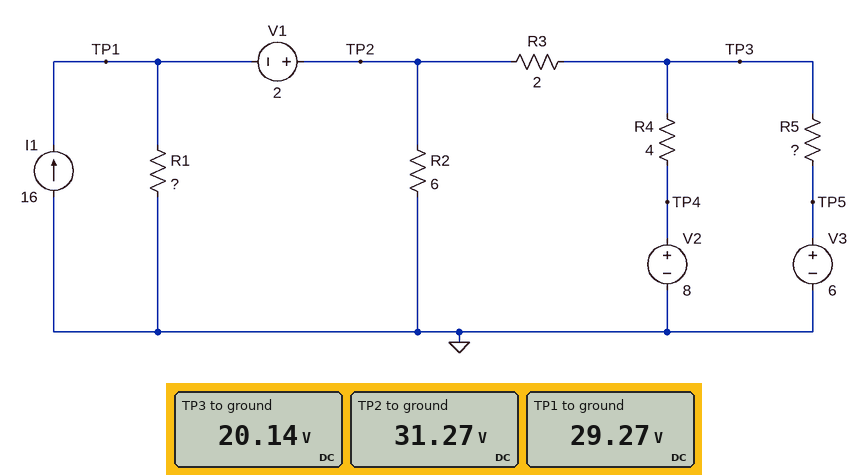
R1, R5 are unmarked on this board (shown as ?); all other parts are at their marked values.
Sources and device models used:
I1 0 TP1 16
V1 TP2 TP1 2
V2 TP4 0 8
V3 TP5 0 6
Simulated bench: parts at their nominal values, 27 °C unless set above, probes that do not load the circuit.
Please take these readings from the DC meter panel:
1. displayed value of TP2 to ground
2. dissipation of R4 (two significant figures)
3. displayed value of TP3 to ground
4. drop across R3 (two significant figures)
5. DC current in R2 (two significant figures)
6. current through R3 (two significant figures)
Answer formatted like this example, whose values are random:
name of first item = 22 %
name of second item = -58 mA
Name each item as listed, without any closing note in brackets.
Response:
displayed value of TP2 to ground = 31.27 V
dissipation of R4 = 37 W
displayed value of TP3 to ground = 20.14 V
drop across R3 = 11 V
DC current in R2 = 5.2 A
current through R3 = 5.6 A
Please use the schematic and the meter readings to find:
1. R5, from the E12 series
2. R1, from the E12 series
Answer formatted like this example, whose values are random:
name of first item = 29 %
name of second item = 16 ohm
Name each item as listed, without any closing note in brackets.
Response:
R5, from the E12 series = 5.6 Ω
R1, from the E12 series = 5.6 Ω
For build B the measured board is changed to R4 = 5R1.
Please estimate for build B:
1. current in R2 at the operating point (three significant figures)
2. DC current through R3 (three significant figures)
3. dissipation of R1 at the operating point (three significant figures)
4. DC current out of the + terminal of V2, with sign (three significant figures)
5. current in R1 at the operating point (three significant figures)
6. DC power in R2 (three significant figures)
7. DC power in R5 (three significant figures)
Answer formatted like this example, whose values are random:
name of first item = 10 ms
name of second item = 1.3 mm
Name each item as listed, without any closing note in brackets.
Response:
current in R2 at the operating point = 5.32 A
DC current through R3 = 5.33 A
dissipation of R1 at the operating point = 160 W
DC current out of the + terminal of V2, with sign = -2.60 A
current in R1 at the operating point = 5.35 A
DC power in R2 = 170 W
DC power in R5 = 41.7 W
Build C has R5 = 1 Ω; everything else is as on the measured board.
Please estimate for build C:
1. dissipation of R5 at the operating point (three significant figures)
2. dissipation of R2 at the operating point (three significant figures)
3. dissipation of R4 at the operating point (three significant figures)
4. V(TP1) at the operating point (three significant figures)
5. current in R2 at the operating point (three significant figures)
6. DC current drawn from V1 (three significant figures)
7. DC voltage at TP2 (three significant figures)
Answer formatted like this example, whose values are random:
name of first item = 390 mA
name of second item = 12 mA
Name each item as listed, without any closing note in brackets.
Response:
dissipation of R5 at the operating point = 37.9 W
dissipation of R2 at the operating point = 117 W
dissipation of R4 at the operating point = 4.32 W
V(TP1) at the operating point = 24.5 V
current in R2 at the operating point = 4.42 A
DC current drawn from V1 = 11.6 A
DC voltage at TP2 = 26.5 V
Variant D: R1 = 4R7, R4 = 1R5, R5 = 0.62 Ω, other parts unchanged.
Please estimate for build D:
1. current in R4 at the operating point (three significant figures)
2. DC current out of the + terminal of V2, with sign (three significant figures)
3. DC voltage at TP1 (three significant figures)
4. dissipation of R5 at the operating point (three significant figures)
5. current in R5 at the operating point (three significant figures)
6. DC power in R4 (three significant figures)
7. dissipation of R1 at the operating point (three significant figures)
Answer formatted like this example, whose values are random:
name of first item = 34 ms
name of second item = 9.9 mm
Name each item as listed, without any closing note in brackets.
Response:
current in R4 at the operating point = 1.17 A
DC current out of the + terminal of V2, with sign = -1.17 A
DC voltage at TP1 = 22.2 V
dissipation of R5 at the operating point = 22.8 W
current in R5 at the operating point = 6.06 A
DC power in R4 = 2.06 W
dissipation of R1 at the operating point = 105 W
